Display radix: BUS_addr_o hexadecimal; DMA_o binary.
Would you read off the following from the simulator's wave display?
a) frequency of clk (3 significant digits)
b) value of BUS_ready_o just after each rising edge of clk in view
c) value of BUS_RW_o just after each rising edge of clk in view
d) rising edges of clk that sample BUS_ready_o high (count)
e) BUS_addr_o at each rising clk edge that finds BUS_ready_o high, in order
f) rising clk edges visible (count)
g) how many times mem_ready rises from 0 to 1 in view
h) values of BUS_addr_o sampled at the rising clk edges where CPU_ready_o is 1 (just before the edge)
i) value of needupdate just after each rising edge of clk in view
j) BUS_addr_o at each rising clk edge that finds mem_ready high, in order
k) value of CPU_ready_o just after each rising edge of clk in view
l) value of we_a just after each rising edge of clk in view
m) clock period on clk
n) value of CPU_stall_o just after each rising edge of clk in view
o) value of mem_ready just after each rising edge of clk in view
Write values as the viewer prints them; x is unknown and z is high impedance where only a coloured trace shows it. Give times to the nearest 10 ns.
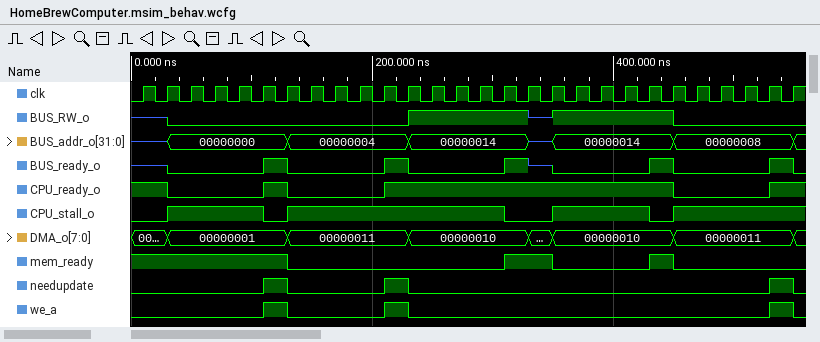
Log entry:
50.0 MHz
z 0 0 0 0 1 0 0 0 0 1 0 0 0 0 1 z 0 0 0 0 1 0 0 0 0 1 0
z 0 0 0 0 0 0 0 0 0 0 1 1 1 1 1 z 1 1 1 1 1 0 0 0 0 0 0
5
00000000, 00000004, 00000014, 00000014, 00000008
28
2
z, z, 00000000, 00000004, 00000014, 00000014, 00000014, 00000014, 00000014, z, 00000014, 00000014, 00000014, 00000014, 00000014, 00000008
0 0 0 0 0 1 0 0 0 0 1 0 0 0 0 0 0 0 0 0 0 0 0 0 0 0 1 0
z, z, 00000000, 00000000, 00000000, 00000000, 00000000, 00000014, z, 00000014
1 0 0 0 0 1 0 0 0 0 1 1 1 1 1 1 1 1 1 1 1 1 0 0 0 0 1 1
0 0 0 0 0 1 0 0 0 0 1 0 0 0 0 0 0 0 0 0 0 0 0 0 0 0 1 0
20 ns
0 1 1 1 1 0 1 1 1 1 1 1 1 1 1 0 0 1 1 1 1 0 1 1 1 1 1 1
1 1 1 1 1 1 0 0 0 0 0 0 0 0 0 1 1 0 0 0 0 1 0 0 0 0 0 0
